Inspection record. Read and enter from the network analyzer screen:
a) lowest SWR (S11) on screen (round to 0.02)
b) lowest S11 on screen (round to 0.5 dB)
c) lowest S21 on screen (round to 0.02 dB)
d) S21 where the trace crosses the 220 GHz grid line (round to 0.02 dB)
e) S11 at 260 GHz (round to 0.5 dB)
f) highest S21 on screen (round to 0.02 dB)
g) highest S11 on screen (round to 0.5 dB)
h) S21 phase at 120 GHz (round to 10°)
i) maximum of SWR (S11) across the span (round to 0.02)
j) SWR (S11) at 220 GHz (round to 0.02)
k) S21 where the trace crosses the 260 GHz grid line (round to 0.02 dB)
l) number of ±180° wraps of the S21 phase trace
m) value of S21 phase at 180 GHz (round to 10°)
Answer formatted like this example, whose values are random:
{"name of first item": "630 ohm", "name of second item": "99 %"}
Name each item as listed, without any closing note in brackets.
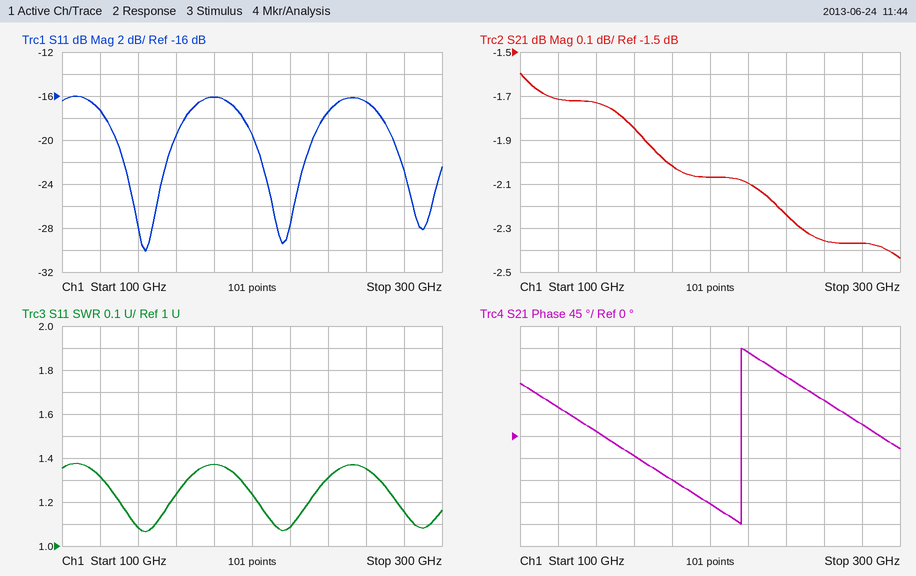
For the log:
{"lowest SWR (S11) on screen": "1.06", "lowest S11 on screen": "-30.0 dB", "lowest S21 on screen": "-2.44 dB", "S21 where the trace crosses the 220 GHz grid line": "-2.10 dB", "S11 at 260 GHz": "-16.5 dB", "highest S21 on screen": "-1.60 dB", "highest S11 on screen": "-16.0 dB", "S21 phase at 120 GHz": "60°", "maximum of SWR (S11) across the span": "1.38", "SWR (S11) at 220 GHz": "1.08", "S21 where the trace crosses the 260 GHz grid line": "-2.36 dB", "number of ±180° wraps of the S21 phase trace": "1", "value of S21 phase at 180 GHz": "-90°"}
